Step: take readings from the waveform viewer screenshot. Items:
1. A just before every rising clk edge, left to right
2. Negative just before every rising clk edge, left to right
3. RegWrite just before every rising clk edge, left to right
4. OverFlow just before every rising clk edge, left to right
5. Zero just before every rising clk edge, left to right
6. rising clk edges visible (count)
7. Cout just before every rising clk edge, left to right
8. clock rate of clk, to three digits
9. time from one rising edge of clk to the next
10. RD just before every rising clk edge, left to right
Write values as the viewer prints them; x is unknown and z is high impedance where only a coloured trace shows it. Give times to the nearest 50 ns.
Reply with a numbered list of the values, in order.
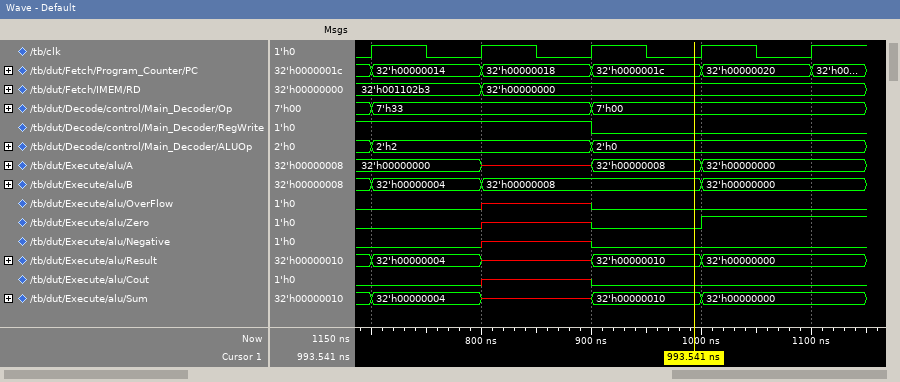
1. 32'h00000000, 32'h00000000, x, 32'h00000008, 32'h00000000
2. 0 0 x 0 0
3. 1 1 1 0 0
4. 0 0 x 0 0
5. 0 0 x 0 1
6. 5
7. 0 0 x 0 0
8. 10.0 MHz
9. 100 ns
10. 32'h001102b3, 32'h001102b3, 32'h00000000, 32'h00000000, 32'h00000000
